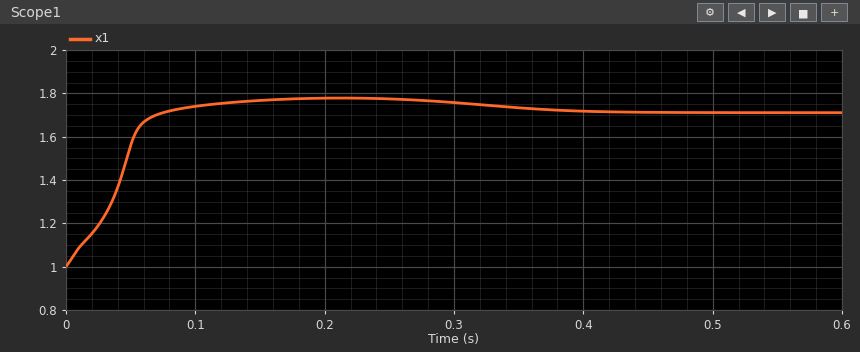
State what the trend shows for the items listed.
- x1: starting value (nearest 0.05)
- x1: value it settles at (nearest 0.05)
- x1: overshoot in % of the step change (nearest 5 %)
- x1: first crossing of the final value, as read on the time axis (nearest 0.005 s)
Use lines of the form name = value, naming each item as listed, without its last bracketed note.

x1: starting value = 1.00
x1: value it settles at = 1.70
x1: overshoot in % of the step change = 10 %
x1: first crossing of the final value, as read on the time axis = 0.075 s
